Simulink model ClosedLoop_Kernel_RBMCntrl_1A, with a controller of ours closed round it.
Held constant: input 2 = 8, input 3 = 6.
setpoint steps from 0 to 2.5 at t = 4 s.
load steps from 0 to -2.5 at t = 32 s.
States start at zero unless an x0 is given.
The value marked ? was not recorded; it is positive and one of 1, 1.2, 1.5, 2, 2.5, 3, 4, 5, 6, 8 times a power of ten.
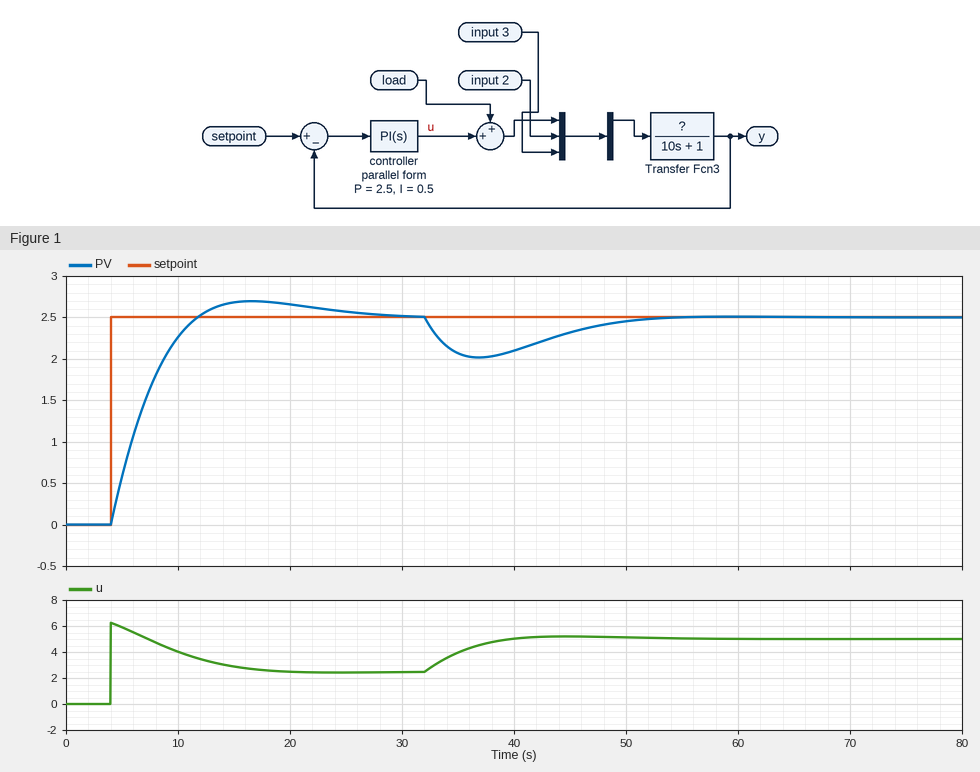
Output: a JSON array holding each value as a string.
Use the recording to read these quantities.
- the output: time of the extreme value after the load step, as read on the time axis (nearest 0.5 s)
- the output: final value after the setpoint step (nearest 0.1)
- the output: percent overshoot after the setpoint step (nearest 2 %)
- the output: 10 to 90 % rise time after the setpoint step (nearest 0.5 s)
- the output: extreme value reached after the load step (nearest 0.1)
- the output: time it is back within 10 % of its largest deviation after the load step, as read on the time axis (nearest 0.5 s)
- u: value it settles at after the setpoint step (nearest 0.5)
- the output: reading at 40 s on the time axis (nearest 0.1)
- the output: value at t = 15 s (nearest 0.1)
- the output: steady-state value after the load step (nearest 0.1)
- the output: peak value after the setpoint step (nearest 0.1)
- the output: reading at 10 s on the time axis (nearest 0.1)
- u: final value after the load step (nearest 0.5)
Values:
["37.0 s", "2.5", "8 %", "5.5 s", "2.0", "50.0 s", "2.5", "2.1", "2.7", "2.5", "2.7", "2.3", "5.0"]
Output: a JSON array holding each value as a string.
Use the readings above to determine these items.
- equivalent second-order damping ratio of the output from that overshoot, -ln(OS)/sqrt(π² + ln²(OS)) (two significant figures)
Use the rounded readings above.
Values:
["0.63"]
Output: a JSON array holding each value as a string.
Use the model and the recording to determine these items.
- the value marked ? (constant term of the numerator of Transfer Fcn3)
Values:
["1"]
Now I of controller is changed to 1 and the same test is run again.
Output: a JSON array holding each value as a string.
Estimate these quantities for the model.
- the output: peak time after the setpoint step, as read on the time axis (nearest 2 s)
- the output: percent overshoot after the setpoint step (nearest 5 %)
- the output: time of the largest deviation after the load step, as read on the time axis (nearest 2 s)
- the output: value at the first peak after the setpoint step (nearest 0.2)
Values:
["12 s", "20 %", "36 s", "3.0"]
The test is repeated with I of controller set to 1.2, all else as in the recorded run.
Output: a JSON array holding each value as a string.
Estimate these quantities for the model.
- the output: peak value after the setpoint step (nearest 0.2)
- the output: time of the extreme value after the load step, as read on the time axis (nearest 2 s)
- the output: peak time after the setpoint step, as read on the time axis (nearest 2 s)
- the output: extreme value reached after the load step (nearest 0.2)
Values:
["3.0", "36 s", "12 s", "2.2"]
